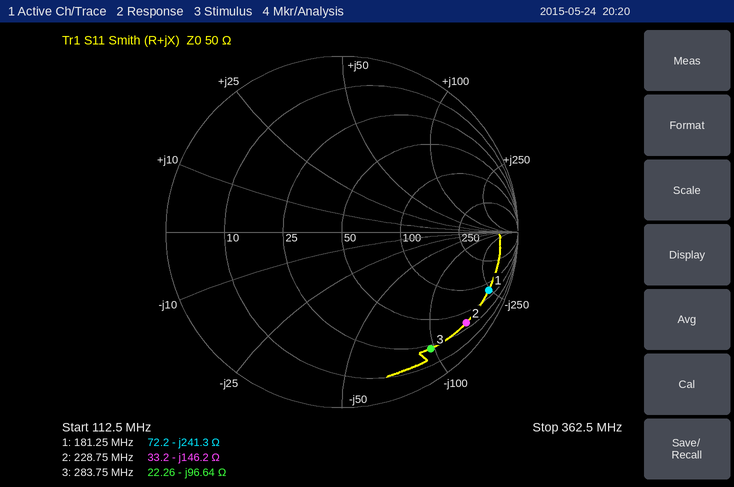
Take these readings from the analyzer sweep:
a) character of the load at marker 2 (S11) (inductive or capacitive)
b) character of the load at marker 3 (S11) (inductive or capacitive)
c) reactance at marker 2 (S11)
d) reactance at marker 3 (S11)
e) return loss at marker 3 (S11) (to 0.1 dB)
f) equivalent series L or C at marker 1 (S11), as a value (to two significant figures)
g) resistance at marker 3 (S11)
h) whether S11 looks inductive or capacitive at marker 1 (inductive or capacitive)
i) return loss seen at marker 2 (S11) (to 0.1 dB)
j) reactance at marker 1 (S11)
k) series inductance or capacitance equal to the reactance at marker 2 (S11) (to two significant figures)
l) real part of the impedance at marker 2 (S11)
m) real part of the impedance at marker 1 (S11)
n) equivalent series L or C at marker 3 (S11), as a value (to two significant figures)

capacitive
capacitive
-146.2 Ω
-96.64 Ω
1.6 dB
3.6 pF
22.26 Ω
capacitive
1.2 dB
-241.3 Ω
4.8 pF
33.2 Ω
72.2 Ω
5.8 pF
